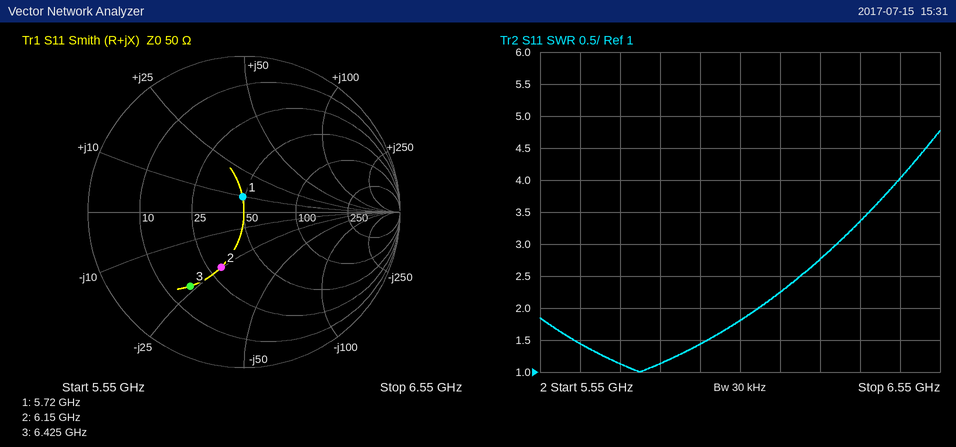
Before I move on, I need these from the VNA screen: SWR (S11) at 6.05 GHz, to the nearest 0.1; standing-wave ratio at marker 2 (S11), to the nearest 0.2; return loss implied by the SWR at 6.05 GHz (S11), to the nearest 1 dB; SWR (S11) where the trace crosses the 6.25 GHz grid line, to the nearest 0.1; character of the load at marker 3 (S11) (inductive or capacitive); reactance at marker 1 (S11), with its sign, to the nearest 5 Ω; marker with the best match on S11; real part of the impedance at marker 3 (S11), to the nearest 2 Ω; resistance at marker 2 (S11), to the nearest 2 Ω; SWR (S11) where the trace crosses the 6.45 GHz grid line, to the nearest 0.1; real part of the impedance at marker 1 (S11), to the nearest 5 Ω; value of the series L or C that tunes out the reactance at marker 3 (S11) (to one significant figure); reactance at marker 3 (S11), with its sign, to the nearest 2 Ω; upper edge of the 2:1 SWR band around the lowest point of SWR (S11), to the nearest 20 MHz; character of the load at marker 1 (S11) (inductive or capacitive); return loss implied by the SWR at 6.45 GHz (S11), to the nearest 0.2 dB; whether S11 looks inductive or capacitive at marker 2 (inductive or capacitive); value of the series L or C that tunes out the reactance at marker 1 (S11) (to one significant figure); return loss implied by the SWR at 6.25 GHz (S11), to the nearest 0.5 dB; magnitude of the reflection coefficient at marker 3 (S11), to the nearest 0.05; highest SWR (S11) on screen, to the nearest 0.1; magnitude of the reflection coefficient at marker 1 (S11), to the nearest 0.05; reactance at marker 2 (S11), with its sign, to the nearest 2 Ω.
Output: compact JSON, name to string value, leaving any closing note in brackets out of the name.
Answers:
{"SWR (S11) at 6.05 GHz, to the nearest 0.1": "1.8", "standing-wave ratio at marker 2 (S11), to the nearest 0.2": "2.2", "return loss implied by the SWR at 6.05 GHz (S11), to the nearest 1 dB": "11 dB", "SWR (S11) where the trace crosses the 6.25 GHz grid line, to the nearest 0.1": "2.8", "character of the load at marker 3 (S11)": "capacitive", "reactance at marker 1 (S11), with its sign, to the nearest 5 Ω": "+10 Ω", "marker with the best match on S11": "marker 1", "real part of the impedance at marker 3 (S11), to the nearest 2 Ω": "16 Ω", "resistance at marker 2 (S11), to the nearest 2 Ω": "30 Ω", "SWR (S11) where the trace crosses the 6.45 GHz grid line, to the nearest 0.1": "4.0", "real part of the impedance at marker 1 (S11), to the nearest 5 Ω": "50 Ω", "value of the series L or C that tunes out the reactance at marker 3 (S11)": "600 pH", "reactance at marker 3 (S11), with its sign, to the nearest 2 Ω": "-24 Ω", "upper edge of the 2:1 SWR band around the lowest point of SWR (S11), to the nearest 20 MHz": "6.10 GHz", "character of the load at marker 1 (S11)": "inductive", "return loss implied by the SWR at 6.45 GHz (S11), to the nearest 0.2 dB": "4.4 dB", "whether S11 looks inductive or capacitive at marker 2": "capacitive", "value of the series L or C that tunes out the reactance at marker 1 (S11)": "3 pF", "return loss implied by the SWR at 6.25 GHz (S11), to the nearest 0.5 dB": "6.5 dB", "magnitude of the reflection coefficient at marker 3 (S11), to the nearest 0.05": "0.60", "highest SWR (S11) on screen, to the nearest 0.1": "4.8", "magnitude of the reflection coefficient at marker 1 (S11), to the nearest 0.05": "0.10", "reactance at marker 2 (S11), with its sign, to the nearest 2 Ω": "-24 Ω"}
